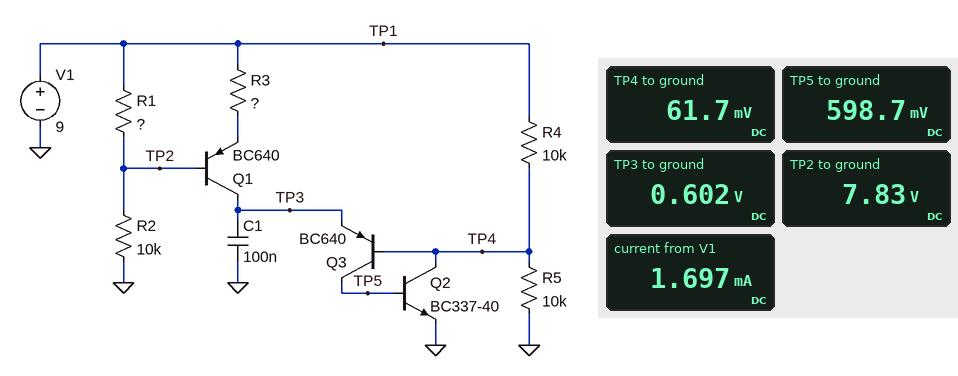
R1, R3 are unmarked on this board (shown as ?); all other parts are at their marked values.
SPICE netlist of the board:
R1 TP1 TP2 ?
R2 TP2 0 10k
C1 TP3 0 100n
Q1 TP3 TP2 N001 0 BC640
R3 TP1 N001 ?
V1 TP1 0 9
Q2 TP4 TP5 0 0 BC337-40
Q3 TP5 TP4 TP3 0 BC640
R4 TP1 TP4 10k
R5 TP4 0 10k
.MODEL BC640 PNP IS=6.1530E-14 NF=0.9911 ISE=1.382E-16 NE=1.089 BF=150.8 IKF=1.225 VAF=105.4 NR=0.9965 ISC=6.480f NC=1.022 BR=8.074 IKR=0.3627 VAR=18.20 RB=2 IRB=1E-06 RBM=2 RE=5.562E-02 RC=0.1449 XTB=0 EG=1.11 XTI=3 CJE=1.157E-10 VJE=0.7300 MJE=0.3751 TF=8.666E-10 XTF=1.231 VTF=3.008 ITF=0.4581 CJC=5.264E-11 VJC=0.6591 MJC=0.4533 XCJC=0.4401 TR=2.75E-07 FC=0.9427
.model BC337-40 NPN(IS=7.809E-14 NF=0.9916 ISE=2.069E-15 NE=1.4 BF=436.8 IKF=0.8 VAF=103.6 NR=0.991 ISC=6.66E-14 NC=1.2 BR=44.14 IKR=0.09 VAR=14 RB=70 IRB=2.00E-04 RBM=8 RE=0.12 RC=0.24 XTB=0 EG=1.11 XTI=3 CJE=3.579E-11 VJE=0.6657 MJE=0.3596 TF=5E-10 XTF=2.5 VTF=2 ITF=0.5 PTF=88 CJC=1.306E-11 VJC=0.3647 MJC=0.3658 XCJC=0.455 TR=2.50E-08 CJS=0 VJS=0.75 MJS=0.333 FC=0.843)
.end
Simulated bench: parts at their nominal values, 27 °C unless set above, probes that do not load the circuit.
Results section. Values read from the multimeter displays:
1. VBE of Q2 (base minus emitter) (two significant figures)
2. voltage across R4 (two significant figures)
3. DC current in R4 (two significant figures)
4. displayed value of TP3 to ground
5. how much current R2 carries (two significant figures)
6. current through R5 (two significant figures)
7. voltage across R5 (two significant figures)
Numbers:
600 mV
8.9 V
890 µA
0.602 V
780 µA
6.2 µA
62 mV
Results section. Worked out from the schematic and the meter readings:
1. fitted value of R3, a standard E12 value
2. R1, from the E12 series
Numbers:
33 kΩ
1.5 kΩ
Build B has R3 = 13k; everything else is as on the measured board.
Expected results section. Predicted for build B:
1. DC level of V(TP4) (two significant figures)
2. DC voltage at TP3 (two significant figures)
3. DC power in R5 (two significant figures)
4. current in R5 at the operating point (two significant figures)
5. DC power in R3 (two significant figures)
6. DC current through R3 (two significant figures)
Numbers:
41 mV
610 mV
170 nW
4.1 µA
32 µW
50 µA
